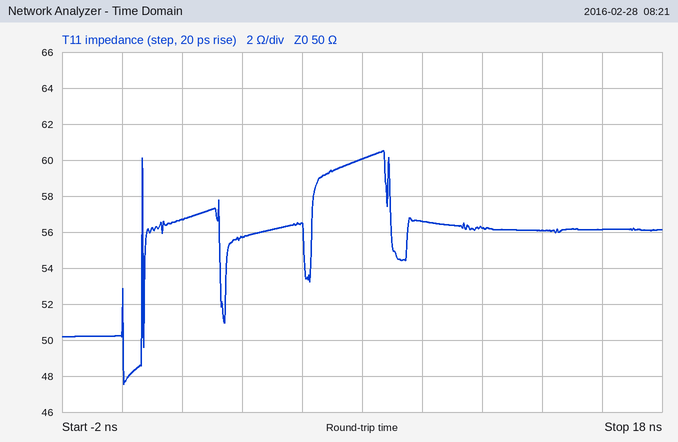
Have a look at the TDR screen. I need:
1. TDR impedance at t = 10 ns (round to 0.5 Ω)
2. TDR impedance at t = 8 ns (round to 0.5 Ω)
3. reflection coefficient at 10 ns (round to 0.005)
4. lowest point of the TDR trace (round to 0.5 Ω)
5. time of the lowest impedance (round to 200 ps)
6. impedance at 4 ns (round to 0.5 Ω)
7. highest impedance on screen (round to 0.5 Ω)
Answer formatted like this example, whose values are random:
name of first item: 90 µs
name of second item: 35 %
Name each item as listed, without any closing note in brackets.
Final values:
TDR impedance at t = 10 ns: 56.5 Ω
TDR impedance at t = 8 ns: 60.0 Ω
reflection coefficient at 10 ns: +0.060
lowest point of the TDR trace: 47.5 Ω
time of the lowest impedance: 0.0 ns
impedance at 4 ns: 55.5 Ω
highest impedance on screen: 60.5 Ω
